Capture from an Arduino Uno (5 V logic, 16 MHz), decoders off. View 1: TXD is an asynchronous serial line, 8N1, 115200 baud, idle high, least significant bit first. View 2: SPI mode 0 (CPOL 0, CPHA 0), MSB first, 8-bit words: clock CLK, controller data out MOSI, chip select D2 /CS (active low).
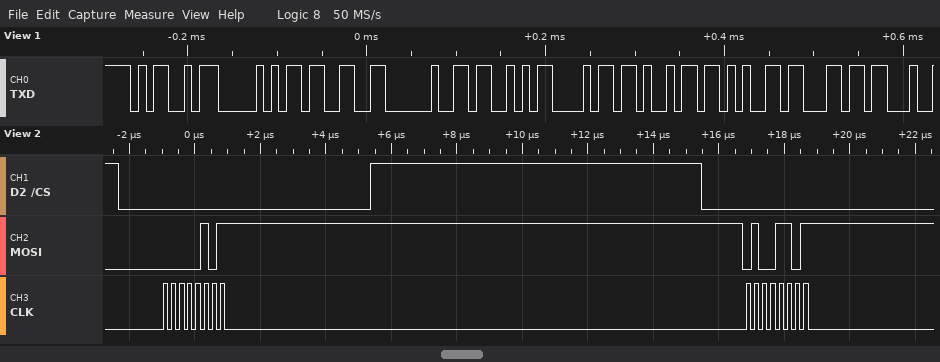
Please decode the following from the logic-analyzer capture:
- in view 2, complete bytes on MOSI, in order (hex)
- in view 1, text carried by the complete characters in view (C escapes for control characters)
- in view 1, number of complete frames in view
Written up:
0x05 0x4D
"MP3 Shiel"
9
